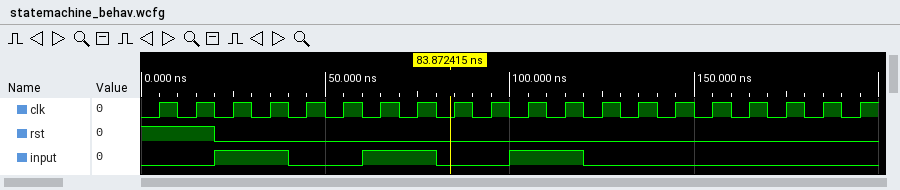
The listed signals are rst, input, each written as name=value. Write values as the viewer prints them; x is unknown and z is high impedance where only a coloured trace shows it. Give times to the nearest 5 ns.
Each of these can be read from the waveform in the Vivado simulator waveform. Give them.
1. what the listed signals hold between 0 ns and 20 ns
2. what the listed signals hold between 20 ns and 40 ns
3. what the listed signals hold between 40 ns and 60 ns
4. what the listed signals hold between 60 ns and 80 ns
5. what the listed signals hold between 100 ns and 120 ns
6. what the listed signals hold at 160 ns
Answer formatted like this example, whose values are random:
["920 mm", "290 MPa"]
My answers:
["rst=1, input=0", "rst=0, input=1", "rst=0, input=0", "rst=0, input=1", "rst=0, input=1", "rst=0, input=0"]
